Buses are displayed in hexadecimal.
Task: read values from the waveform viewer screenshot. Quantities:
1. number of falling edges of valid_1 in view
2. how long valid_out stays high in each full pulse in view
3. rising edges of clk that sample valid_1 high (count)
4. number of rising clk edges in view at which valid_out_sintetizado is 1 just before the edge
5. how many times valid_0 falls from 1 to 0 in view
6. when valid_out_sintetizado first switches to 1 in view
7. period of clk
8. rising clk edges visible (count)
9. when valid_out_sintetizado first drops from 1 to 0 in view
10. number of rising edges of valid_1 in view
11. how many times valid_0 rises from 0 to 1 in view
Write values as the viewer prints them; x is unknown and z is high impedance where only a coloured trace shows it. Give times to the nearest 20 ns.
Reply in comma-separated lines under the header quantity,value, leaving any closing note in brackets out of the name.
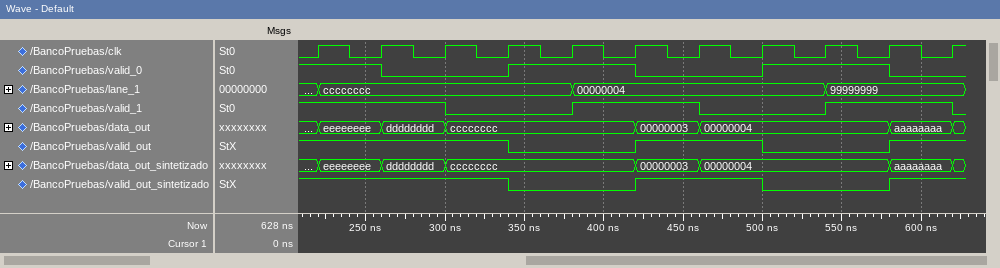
quantity,value
number of falling edges of valid_1 in view,3
how long valid_out stays high in each full pulse in view,80 ns
rising edges of clk that sample valid_1 high,7
number of rising clk edges in view at which valid_out_sintetizado is 1 just before the edge,7
how many times valid_0 falls from 1 to 0 in view,3
when valid_out_sintetizado first switches to 1 in view,420 ns
period of clk,40 ns
rising clk edges visible,11
when valid_out_sintetizado first drops from 1 to 0 in view,340 ns
number of rising edges of valid_1 in view,2
how many times valid_0 rises from 0 to 1 in view,2
